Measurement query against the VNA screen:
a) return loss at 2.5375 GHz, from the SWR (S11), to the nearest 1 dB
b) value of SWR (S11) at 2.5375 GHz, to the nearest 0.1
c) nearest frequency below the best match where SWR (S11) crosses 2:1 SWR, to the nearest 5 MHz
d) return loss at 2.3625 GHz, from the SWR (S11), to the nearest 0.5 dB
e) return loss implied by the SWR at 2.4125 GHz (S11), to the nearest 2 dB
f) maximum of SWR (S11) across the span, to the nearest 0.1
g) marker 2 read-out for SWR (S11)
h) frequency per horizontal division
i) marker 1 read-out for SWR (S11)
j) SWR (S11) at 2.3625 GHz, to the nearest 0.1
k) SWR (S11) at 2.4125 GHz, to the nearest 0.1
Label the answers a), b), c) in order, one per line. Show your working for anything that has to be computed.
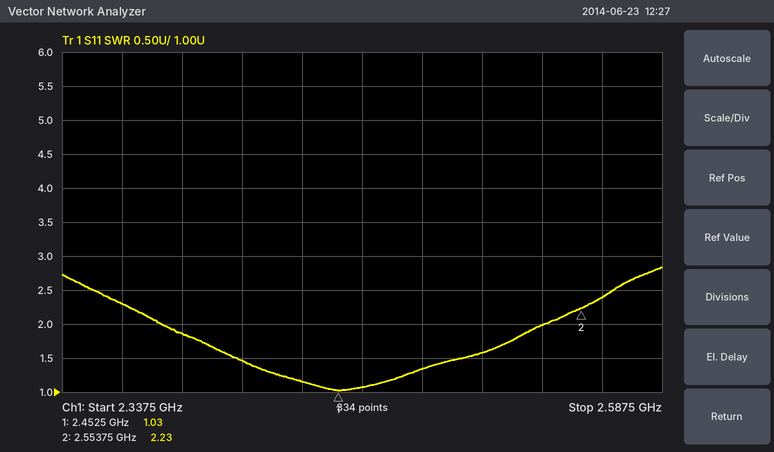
a) −20 log10((2 − 1)/(2 + 1)) ≈ 10 dB
b) 2.0
c) 2.380 GHz
d) −20 log10((2.3 − 1)/(2.3 + 1)) ≈ 8.09 dB, so 8.0 dB to the nearest 0.5 dB
e) −20 log10((1.5 − 1)/(1.5 + 1)) ≈ 14 dB
f) 2.8
g) 2.23
h) 25 MHz
i) 1.03
j) 2.3
k) 1.5
